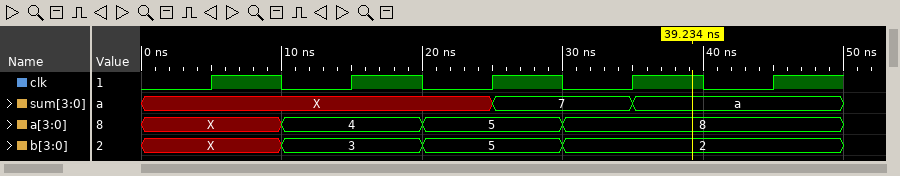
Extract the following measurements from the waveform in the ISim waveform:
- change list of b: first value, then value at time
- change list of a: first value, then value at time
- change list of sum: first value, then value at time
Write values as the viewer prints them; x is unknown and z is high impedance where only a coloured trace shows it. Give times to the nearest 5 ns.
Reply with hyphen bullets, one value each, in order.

- X, 3 at 10 ns, 5 at 20 ns, 2 at 30 ns
- X, 4 at 10 ns, 5 at 20 ns, 8 at 30 ns
- X, 7 at 25 ns, a at 35 ns
